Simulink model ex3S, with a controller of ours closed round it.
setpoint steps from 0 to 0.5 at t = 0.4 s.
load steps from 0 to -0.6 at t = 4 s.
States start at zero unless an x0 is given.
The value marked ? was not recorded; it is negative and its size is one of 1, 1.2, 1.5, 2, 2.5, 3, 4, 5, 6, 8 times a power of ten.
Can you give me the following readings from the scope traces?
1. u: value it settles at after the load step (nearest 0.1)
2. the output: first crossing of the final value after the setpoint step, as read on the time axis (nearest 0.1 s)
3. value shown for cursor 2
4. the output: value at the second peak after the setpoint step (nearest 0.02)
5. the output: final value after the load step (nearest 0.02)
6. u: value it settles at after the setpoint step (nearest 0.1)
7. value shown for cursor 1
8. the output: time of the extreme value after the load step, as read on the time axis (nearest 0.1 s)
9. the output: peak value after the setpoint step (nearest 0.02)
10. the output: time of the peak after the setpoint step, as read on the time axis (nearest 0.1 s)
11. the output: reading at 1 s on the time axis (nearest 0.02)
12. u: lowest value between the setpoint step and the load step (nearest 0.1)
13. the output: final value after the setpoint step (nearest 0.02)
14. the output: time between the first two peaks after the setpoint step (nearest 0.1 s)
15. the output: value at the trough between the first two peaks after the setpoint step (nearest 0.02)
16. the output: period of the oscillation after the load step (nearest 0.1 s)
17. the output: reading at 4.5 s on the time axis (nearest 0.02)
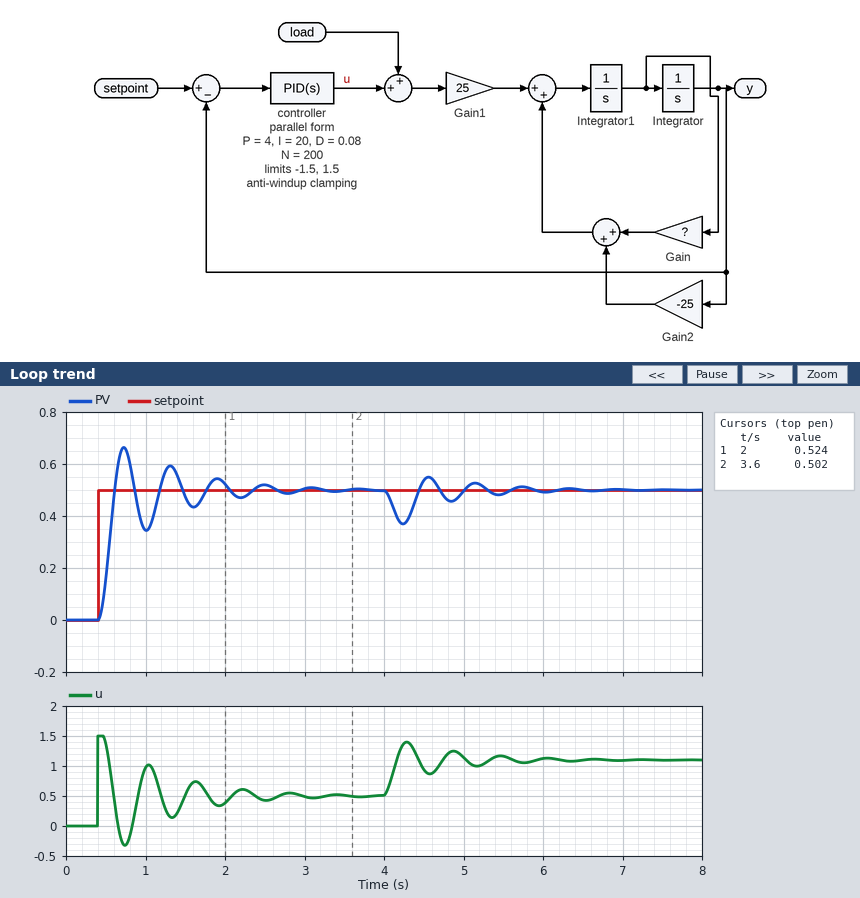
1.1
0.6 s
0.502
0.60
0.50
0.5
0.524
4.2 s
0.66
0.7 s
0.34
-0.3
0.50
0.6 s
0.34
0.6 s
0.54
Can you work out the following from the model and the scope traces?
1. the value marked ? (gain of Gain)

-5
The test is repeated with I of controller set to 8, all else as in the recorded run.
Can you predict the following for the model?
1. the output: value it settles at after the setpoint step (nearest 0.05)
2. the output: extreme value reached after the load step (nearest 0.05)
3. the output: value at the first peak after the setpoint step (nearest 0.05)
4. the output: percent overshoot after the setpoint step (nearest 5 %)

0.50
0.35
0.60
20 %
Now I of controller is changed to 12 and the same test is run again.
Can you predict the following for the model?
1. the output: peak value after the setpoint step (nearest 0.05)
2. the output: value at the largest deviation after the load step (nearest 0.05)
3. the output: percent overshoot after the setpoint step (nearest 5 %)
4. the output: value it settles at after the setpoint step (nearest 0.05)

0.60
0.35
25 %
0.50
